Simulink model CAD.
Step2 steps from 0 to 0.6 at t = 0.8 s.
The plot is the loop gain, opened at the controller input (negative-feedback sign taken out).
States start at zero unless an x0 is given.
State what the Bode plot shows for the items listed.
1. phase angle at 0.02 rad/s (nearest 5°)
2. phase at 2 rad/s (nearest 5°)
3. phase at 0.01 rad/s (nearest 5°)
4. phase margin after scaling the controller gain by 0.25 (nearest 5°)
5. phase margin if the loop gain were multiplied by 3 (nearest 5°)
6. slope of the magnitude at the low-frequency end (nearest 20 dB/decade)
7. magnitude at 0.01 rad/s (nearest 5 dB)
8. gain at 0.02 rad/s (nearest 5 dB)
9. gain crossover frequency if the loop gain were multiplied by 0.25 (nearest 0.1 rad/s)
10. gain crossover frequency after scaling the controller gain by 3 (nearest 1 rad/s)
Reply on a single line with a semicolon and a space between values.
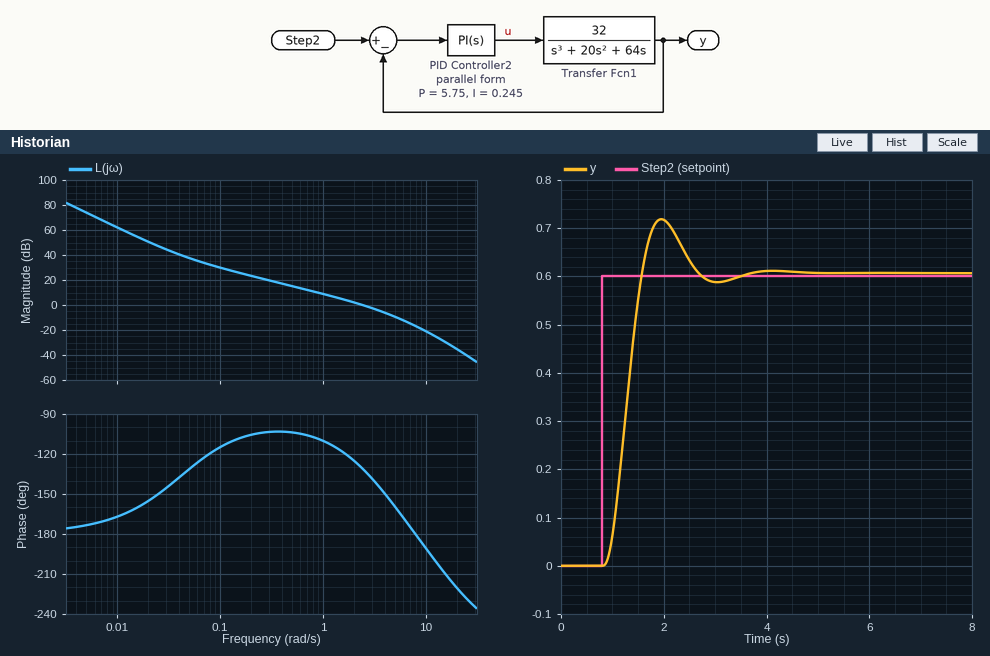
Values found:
-155°; -125°; -165°; 75°; 20°; -40 dB/decade; 60 dB; 50 dB; 0.7 rad/s; 5 rad/s
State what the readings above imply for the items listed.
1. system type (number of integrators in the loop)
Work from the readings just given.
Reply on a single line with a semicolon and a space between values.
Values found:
2
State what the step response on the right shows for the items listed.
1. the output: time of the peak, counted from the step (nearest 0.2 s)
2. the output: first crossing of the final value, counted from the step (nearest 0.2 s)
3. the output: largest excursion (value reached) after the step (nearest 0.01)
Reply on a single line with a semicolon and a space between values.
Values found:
1.2 s; 0.8 s; 0.72
